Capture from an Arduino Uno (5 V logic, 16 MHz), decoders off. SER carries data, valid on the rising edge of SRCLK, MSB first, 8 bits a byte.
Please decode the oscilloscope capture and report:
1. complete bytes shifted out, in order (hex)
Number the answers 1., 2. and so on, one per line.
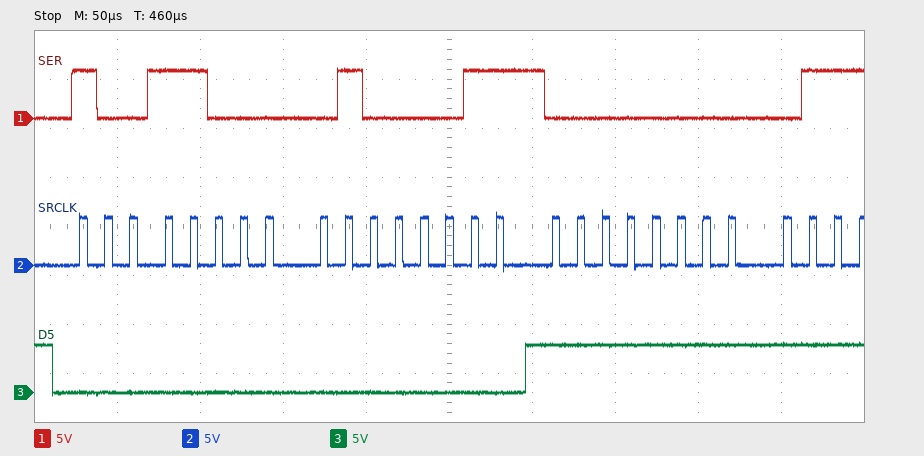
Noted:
1. 98 43 00
